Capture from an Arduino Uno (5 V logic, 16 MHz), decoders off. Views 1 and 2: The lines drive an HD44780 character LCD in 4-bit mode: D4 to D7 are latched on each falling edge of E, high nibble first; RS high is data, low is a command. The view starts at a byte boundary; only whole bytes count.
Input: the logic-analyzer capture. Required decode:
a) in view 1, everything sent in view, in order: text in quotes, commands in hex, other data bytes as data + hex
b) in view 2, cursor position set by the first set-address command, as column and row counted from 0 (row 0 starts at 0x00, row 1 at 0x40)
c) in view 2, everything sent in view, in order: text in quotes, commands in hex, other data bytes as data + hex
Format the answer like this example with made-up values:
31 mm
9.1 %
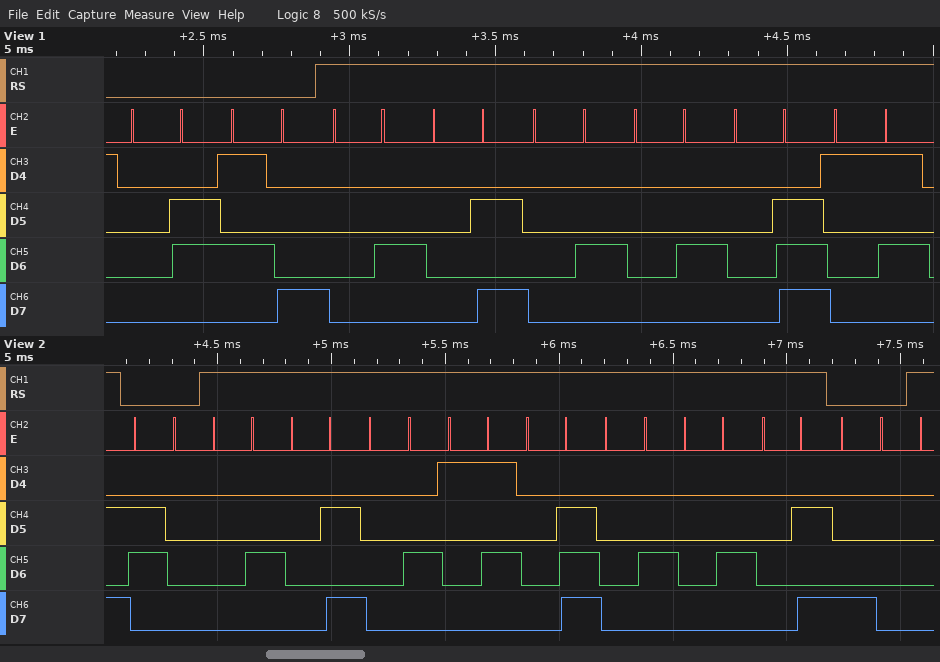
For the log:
0x06 0x58 data 04 0A 04 04 0E 15
column 0, row 0
0x60 data 04 0A 04 15 0E 04 04 0A 0x80
